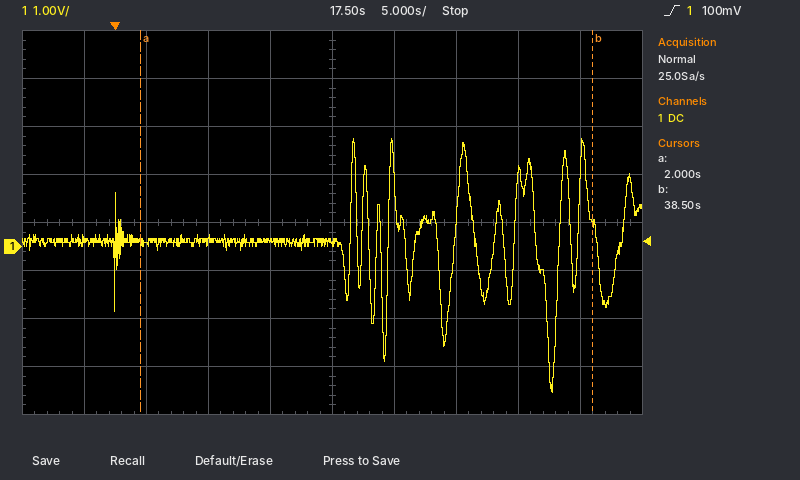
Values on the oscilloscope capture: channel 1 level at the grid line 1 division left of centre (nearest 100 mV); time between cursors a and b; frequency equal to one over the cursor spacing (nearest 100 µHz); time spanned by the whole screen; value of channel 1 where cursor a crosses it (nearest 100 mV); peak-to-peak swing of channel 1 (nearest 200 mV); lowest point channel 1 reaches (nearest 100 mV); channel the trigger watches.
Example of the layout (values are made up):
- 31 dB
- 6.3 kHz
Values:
- 100 mV
- 36.5 s
- 27.4 mHz
- 50 s
- 100 mV
- 5.2 V
- -3.0 V
- channel 1
